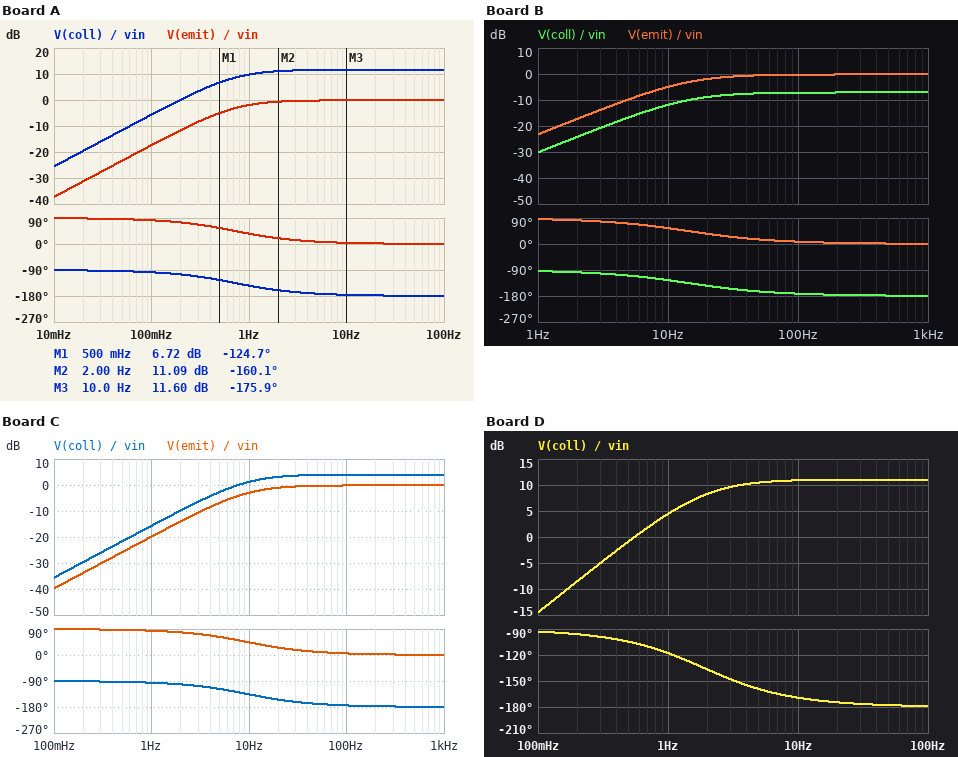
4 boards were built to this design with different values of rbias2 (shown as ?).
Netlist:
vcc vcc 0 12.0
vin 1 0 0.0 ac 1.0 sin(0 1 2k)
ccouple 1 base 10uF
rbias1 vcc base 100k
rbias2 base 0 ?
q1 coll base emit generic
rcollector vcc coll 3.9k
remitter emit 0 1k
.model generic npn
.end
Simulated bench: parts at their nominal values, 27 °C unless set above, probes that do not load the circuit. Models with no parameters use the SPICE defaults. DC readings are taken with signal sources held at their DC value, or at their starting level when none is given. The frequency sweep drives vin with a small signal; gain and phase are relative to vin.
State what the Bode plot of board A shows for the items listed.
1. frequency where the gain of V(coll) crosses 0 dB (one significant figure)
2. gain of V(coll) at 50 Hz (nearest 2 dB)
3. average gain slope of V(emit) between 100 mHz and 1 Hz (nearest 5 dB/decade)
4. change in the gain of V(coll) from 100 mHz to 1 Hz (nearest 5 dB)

200 mHz
12 dB
15 dB/decade
15 dB
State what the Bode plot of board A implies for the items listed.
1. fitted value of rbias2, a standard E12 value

39 kΩ
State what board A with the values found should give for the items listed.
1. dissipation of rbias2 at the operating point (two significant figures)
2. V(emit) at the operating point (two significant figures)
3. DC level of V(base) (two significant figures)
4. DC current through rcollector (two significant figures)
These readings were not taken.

200 µW
2.0 V
2.8 V
2.0 mA
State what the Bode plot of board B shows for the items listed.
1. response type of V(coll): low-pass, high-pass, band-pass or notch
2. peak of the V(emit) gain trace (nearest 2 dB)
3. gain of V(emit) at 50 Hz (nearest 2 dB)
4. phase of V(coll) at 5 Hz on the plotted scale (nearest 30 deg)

high-pass
0 dB
0 dB
-120 deg
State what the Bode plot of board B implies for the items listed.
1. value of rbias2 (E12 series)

68 kΩ
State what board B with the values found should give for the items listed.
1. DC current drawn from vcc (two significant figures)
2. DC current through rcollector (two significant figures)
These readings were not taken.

2.5 mA
2.4 mA
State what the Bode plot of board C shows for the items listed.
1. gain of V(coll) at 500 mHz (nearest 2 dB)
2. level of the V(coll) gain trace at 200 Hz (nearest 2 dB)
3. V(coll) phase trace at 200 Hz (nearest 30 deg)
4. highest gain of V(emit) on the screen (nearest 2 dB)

-22 dB
4 dB
-180 deg
0 dB
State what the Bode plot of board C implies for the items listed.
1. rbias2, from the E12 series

56 kΩ
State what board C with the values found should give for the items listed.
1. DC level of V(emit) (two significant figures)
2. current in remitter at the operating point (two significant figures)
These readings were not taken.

2.4 V
2.4 mA
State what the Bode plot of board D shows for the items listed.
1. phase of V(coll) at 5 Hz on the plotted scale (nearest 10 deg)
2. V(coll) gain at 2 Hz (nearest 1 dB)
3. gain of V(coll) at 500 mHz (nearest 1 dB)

-160 deg
8 dB
-1 dB
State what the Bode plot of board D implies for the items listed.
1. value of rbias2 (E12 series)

10 kΩ
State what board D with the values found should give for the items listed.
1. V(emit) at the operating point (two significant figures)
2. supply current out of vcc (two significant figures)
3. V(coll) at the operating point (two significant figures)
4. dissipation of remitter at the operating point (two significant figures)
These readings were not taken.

320 mV
420 µA
11 V
100 µW
